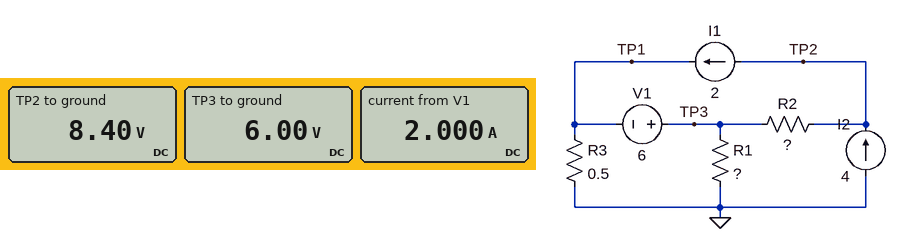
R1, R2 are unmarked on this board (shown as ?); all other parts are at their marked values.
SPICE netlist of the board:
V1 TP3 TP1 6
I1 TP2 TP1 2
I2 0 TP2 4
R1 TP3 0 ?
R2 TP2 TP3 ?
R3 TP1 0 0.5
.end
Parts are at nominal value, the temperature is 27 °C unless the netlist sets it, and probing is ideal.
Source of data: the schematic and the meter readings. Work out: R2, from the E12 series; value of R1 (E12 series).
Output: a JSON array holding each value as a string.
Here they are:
["1.2 Ω", "1.5 Ω"]
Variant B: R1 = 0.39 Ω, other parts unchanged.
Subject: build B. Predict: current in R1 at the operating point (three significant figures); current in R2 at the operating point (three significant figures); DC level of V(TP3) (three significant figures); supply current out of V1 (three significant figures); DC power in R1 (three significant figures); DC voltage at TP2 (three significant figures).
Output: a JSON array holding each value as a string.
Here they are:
["8.99 A", "2.00 A", "3.51 V", "6.99 A", "31.5 W", "5.91 V"]
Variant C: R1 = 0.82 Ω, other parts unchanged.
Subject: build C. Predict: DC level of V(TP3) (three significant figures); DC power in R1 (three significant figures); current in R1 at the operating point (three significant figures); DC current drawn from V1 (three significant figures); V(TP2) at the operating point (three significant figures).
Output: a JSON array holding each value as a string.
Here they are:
["4.97 V", "30.1 W", "6.06 A", "4.06 A", "7.37 V"]
